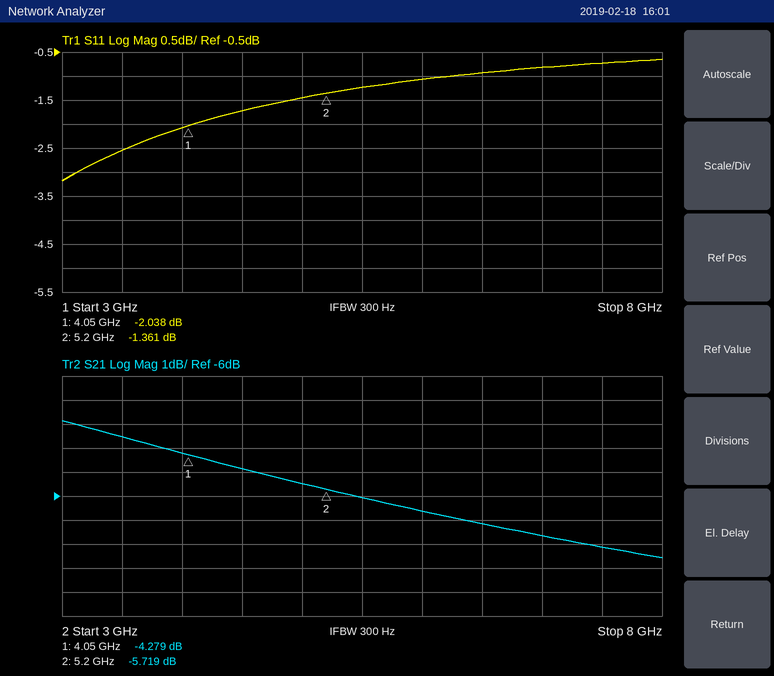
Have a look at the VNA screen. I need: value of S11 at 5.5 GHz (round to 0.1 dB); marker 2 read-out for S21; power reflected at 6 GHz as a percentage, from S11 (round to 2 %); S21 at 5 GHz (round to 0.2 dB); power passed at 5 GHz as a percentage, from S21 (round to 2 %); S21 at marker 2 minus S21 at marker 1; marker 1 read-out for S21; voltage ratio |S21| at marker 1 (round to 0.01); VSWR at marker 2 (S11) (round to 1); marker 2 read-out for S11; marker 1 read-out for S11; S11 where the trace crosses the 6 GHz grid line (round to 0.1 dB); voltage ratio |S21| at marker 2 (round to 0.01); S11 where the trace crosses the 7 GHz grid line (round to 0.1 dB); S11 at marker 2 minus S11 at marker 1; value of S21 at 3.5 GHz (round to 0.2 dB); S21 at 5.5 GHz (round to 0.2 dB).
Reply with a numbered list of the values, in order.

1. -1.2 dB
2. -5.719 dB
3. 78 %
4. -5.4 dB
5. 28 %
6. -1.440 dB
7. -4.279 dB
8. 0.61
9. 13
10. -1.361 dB
11. -2.038 dB
12. -1.1 dB
13. 0.52
14. -0.8 dB
15. 0.677 dB
16. -3.6 dB
17. -6.0 dB
